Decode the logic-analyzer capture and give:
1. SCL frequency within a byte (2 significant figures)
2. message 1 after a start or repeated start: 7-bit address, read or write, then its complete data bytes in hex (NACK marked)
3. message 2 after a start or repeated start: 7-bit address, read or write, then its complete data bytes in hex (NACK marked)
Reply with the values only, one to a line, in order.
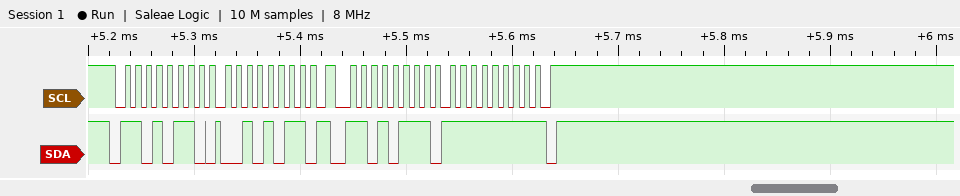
100 kHz
0x6B write: 2B
0x6B read: FF NACK
